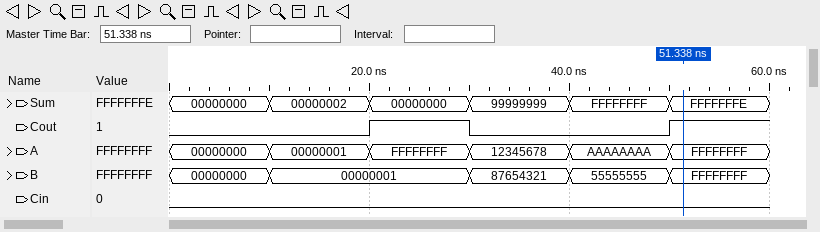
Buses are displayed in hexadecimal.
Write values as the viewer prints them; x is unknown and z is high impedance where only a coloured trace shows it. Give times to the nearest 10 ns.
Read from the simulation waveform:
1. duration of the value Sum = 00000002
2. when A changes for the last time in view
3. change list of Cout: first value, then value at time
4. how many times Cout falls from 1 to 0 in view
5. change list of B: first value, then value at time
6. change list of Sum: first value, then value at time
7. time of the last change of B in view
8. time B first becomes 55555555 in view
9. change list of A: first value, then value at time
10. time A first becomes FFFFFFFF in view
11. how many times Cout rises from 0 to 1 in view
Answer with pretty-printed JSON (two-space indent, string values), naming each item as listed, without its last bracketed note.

{
  "duration of the value Sum = 00000002": "10 ns",
  "when A changes for the last time in view": "50 ns",
  "change list of Cout: first value, then value at time": "0, 1 at 20 ns, 0 at 30 ns, 1 at 50 ns",
  "how many times Cout falls from 1 to 0 in view": "1",
  "change list of B: first value, then value at time": "00000000, 00000001 at 10 ns, 87654321 at 30 ns, 55555555 at 40 ns, FFFFFFFF at 50 ns",
  "change list of Sum: first value, then value at time": "00000000, 00000002 at 10 ns, 00000000 at 20 ns, 99999999 at 30 ns, FFFFFFFF at 40 ns, FFFFFFFE at 50 ns",
  "time of the last change of B in view": "50 ns",
  "time B first becomes 55555555 in view": "40 ns",
  "change list of A: first value, then value at time": "00000000, 00000001 at 10 ns, FFFFFFFF at 20 ns, 12345678 at 30 ns, AAAAAAAA at 40 ns, FFFFFFFF at 50 ns",
  "time A first becomes FFFFFFFF in view": "20 ns",
  "how many times Cout rises from 0 to 1 in view": "2"
}
